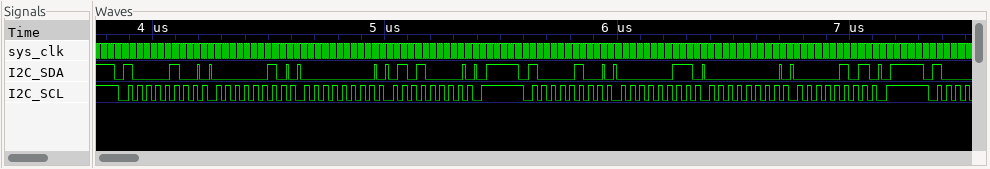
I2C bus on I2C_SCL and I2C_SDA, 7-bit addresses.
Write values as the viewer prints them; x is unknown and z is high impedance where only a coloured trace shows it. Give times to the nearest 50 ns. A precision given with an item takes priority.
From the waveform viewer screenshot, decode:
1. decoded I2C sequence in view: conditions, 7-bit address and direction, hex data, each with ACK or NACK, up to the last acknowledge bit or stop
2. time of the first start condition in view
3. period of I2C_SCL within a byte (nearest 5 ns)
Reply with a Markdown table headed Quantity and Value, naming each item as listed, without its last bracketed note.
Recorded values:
| Quantity | Value |
|---|---|
| decoded I2C sequence in view: conditions, 7-bit address and direction, hex data, each with ACK or NACK, up to the last acknowledge bit or stop | start, address 42 write ACK, 02 ACK, 00 ACK, 50 ACK, stop, start, address 42 write ACK, 03 ACK, 00 ACK, 05 ACK, stop |
| time of the first start condition in view | 3850 ns |
| period of I2C_SCL within a byte | 40 ns |
